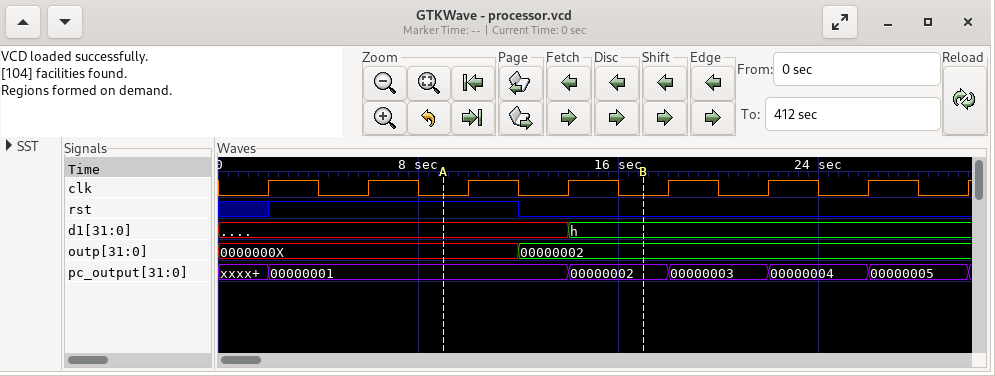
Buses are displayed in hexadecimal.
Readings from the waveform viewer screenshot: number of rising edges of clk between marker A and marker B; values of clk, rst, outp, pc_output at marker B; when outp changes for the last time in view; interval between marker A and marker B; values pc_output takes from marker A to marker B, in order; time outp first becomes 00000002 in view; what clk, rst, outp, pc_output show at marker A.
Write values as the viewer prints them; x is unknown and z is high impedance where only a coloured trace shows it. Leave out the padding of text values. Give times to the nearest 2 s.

2
clk=0, rst=0, outp=00000002, pc_output=00000002
12 s
8 s
00000001, 00000002
12 s
clk=0, rst=1, outp=0000000X, pc_output=00000001
